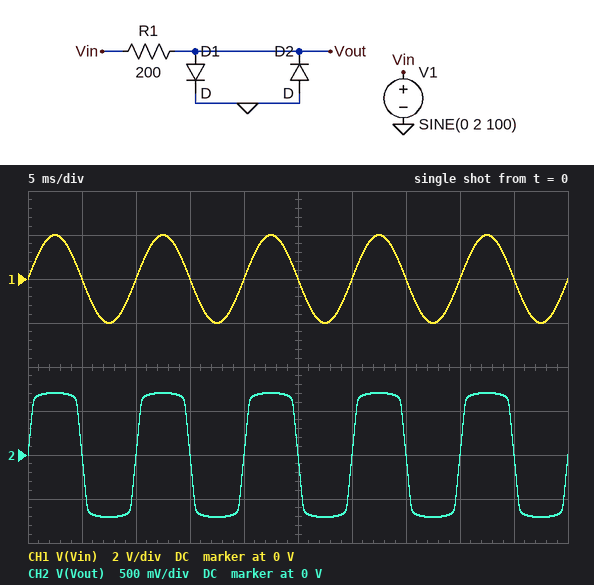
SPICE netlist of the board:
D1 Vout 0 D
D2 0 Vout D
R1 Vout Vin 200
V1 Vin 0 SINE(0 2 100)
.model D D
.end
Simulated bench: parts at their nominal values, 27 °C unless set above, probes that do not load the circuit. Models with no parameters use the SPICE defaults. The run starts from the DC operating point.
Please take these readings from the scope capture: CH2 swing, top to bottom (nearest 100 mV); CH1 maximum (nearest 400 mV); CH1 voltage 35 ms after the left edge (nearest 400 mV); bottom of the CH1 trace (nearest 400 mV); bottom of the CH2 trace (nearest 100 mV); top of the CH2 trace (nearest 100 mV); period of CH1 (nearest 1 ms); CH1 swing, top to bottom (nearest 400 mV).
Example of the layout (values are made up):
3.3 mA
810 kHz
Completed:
1.4 V
2.0 V
0 V
-2.0 V
-700 mV
700 mV
10 ms
4.0 V
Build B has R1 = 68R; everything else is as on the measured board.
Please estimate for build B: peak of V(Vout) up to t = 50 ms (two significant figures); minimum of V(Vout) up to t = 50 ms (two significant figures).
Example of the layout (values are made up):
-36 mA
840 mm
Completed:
730 mV
-730 mV
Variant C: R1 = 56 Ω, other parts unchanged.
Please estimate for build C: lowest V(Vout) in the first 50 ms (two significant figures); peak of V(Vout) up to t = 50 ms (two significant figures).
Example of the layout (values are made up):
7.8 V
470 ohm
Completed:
-740 mV
740 mV
